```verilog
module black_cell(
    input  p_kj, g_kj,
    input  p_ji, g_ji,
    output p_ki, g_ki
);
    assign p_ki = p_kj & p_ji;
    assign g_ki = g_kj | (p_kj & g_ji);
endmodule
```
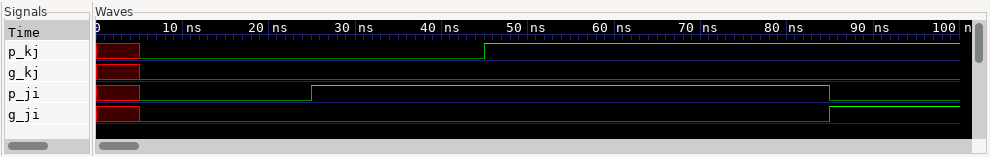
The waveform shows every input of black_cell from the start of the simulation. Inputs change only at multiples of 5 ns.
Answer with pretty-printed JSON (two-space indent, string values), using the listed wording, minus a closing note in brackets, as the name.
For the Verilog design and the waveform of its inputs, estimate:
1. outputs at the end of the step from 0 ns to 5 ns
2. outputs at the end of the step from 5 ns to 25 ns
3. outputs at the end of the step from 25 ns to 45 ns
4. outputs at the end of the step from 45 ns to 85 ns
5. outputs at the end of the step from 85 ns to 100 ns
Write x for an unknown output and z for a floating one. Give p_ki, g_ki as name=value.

{
  "outputs at the end of the step from 0 ns to 5 ns": "p_ki=x, g_ki=x",
  "outputs at the end of the step from 5 ns to 25 ns": "p_ki=0, g_ki=0",
  "outputs at the end of the step from 25 ns to 45 ns": "p_ki=0, g_ki=0",
  "outputs at the end of the step from 45 ns to 85 ns": "p_ki=1, g_ki=0",
  "outputs at the end of the step from 85 ns to 100 ns": "p_ki=0, g_ki=1"
}
